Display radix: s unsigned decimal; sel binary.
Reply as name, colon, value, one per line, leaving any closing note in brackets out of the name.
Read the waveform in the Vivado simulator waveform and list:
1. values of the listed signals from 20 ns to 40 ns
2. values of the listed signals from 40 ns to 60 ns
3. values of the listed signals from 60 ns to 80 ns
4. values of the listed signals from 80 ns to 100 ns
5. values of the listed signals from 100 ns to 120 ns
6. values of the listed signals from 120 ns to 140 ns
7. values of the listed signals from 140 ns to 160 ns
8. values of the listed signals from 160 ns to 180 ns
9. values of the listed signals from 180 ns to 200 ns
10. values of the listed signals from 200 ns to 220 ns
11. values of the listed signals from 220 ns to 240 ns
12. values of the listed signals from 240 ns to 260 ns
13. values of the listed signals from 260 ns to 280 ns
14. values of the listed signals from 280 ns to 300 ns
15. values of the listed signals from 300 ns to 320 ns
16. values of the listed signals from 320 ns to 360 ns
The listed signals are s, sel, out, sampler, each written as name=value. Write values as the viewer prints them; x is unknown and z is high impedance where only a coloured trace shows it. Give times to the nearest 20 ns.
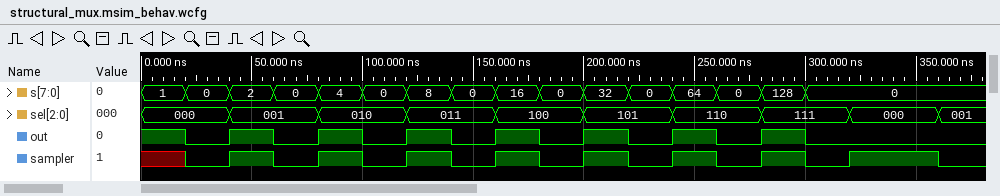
values of the listed signals from 20 ns to 40 ns: s=0, sel=000, out=0, sampler=0
values of the listed signals from 40 ns to 60 ns: s=2, sel=001, out=1, sampler=1
values of the listed signals from 60 ns to 80 ns: s=0, sel=001, out=0, sampler=0
values of the listed signals from 80 ns to 100 ns: s=4, sel=010, out=1, sampler=1
values of the listed signals from 100 ns to 120 ns: s=0, sel=010, out=0, sampler=0
values of the listed signals from 120 ns to 140 ns: s=8, sel=011, out=1, sampler=1
values of the listed signals from 140 ns to 160 ns: s=0, sel=011, out=0, sampler=0
values of the listed signals from 160 ns to 180 ns: s=16, sel=100, out=1, sampler=1
values of the listed signals from 180 ns to 200 ns: s=0, sel=100, out=0, sampler=0
values of the listed signals from 200 ns to 220 ns: s=32, sel=101, out=1, sampler=1
values of the listed signals from 220 ns to 240 ns: s=0, sel=101, out=0, sampler=0
values of the listed signals from 240 ns to 260 ns: s=64, sel=110, out=1, sampler=1
values of the listed signals from 260 ns to 280 ns: s=0, sel=110, out=0, sampler=0
values of the listed signals from 280 ns to 300 ns: s=128, sel=111, out=1, sampler=1
values of the listed signals from 300 ns to 320 ns: s=0, sel=111, out=0, sampler=0
values of the listed signals from 320 ns to 360 ns: s=0, sel=000, out=0, sampler=1
